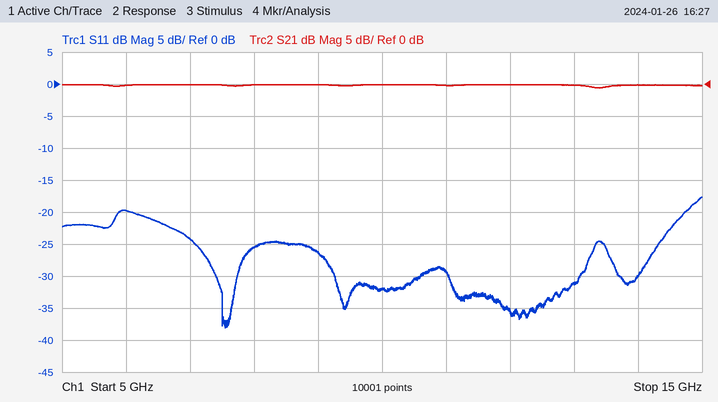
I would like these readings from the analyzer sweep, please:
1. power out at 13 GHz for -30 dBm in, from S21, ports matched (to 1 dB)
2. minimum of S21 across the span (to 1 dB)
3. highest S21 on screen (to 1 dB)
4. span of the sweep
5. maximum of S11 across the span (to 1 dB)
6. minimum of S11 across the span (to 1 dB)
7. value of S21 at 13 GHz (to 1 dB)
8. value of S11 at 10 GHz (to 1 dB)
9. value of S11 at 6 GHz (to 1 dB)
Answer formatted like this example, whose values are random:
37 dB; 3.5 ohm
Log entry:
-30 dBm; -1 dB; 0 dB; 10 GHz; -18 dB; -38 dB; 0 dB; -32 dB; -20 dB
